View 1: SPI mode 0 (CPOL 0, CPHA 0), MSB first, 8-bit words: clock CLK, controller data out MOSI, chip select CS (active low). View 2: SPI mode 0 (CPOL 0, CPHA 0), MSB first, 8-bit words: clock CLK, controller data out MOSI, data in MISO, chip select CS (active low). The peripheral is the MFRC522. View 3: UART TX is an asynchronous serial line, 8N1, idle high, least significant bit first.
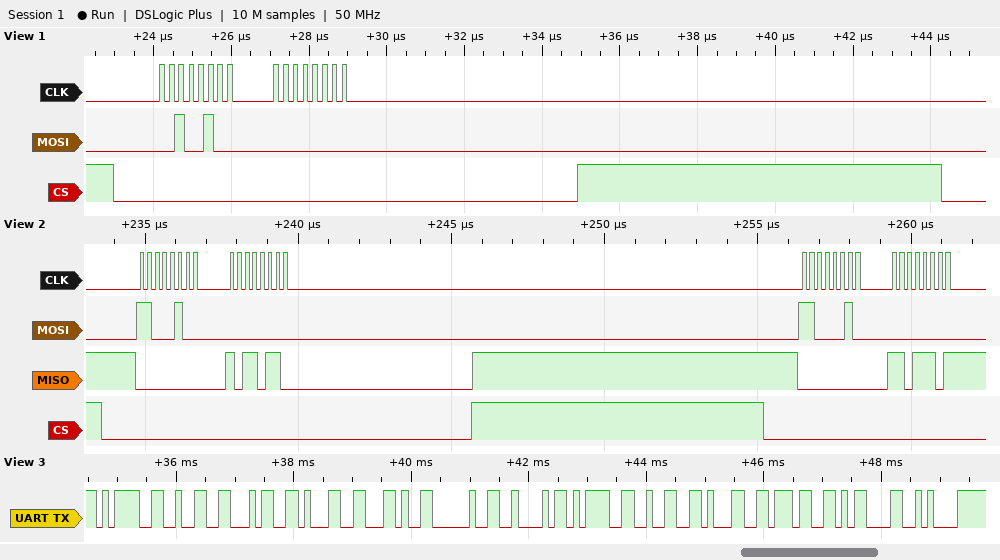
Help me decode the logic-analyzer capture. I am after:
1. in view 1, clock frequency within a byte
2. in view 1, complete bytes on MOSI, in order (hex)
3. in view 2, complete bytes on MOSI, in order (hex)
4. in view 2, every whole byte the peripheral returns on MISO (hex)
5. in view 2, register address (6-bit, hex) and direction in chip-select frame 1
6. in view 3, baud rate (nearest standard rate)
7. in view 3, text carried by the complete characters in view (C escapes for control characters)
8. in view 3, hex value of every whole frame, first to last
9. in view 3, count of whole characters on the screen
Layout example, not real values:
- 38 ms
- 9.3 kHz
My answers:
- 4 MHz
- 0x24 0x00
- C4 00 C2 00
- 00 B6 00 DD
- 0x22 read
- 9600 baud
- "=241, B=217\r\n"
- 3D 32 34 31 2C 20 42 3D 32 31 37 0D 0A
- 13
